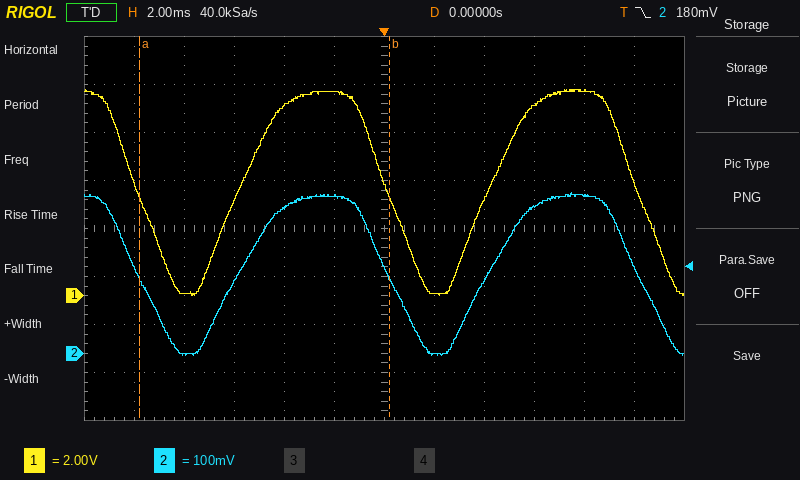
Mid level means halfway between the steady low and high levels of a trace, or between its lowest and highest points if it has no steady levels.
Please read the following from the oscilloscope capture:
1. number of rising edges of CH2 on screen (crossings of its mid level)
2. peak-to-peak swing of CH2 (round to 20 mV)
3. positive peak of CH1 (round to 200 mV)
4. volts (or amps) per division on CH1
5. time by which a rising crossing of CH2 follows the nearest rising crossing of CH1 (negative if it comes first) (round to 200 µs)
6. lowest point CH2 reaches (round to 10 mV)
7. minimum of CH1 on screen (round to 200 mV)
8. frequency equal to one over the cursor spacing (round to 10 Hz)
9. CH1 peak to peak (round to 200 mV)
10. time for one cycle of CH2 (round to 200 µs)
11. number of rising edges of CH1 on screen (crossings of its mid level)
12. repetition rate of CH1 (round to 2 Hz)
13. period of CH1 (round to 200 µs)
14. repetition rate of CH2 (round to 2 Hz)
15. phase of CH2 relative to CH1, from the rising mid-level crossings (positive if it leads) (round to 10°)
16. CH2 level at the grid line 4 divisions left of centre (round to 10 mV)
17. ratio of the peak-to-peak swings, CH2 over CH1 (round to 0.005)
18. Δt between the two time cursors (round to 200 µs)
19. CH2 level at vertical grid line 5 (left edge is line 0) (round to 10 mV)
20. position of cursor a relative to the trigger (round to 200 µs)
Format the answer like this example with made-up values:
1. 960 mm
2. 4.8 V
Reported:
1. 2
2. 340 mV
3. 8.6 V
4. 2 V
5. 0.0 ms
6. 0 mV
7. 0.0 V
8. 100 Hz
9. 8.6 V
10. 10.0 ms
11. 2
12. 100 Hz
13. 10.0 ms
14. 100 Hz
15. 0°
16. 0 mV
17. 0.040
18. 10.0 ms
19. 330 mV
20. -9.8 ms
